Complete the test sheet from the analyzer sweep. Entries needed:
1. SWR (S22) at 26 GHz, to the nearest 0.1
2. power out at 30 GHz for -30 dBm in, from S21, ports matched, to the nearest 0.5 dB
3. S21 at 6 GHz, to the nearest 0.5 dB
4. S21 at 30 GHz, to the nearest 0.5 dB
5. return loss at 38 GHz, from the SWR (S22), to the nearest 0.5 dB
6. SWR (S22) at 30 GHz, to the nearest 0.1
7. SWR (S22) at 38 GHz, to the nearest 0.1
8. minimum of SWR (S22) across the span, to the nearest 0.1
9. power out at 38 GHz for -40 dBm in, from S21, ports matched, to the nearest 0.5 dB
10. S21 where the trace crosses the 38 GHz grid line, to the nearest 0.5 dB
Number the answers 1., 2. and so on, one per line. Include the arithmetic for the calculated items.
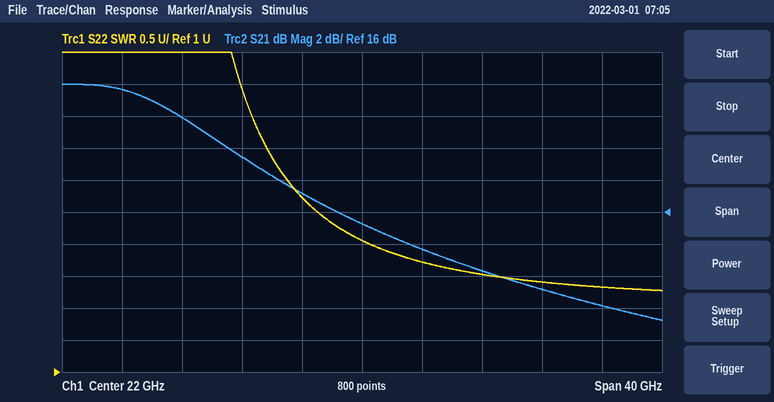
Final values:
1. 2.7
2. -30 dBm + (12.5 dB) = -17.5 dBm
3. 23.5 dB
4. 12.5 dB
5. −20 log10((2.3 − 1)/(2.3 + 1)) ≈ 8.09 dB, so 8.0 dB to the nearest 0.5 dB
6. 2.5
7. 2.3
8. 2.3
9. -40 dBm + (10.0 dB) = -30.0 dBm
10. 10.0 dB
